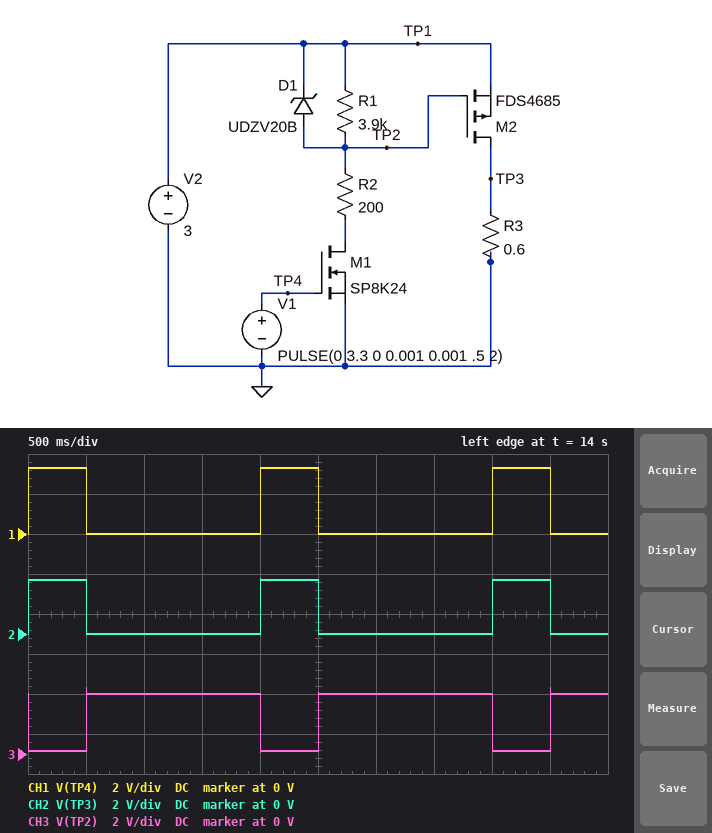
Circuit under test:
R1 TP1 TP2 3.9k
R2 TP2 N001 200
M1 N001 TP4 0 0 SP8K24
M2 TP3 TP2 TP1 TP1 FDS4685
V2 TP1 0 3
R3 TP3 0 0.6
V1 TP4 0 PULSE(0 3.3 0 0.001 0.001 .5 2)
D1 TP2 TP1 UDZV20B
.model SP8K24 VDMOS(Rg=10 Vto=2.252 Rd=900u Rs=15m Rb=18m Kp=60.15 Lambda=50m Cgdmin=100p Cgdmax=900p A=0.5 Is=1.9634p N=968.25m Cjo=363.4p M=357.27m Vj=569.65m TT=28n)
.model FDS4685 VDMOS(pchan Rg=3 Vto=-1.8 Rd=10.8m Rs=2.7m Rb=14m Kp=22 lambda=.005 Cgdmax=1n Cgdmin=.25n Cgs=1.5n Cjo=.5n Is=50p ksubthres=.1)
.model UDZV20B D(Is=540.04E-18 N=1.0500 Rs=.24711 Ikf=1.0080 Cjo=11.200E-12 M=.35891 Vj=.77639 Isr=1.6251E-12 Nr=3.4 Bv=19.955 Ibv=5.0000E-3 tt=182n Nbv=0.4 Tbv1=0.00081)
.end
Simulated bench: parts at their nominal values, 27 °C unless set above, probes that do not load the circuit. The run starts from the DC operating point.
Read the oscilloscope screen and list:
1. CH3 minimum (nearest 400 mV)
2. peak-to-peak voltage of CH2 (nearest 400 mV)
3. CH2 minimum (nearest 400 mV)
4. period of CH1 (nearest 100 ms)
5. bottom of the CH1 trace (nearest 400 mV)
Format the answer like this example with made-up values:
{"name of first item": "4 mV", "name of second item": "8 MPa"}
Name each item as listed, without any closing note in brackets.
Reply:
{"CH3 minimum": "0 V", "peak-to-peak voltage of CH2": "2.8 V", "CH2 minimum": "0 V", "period of CH1": "2.0 s", "bottom of the CH1 trace": "0 V"}
